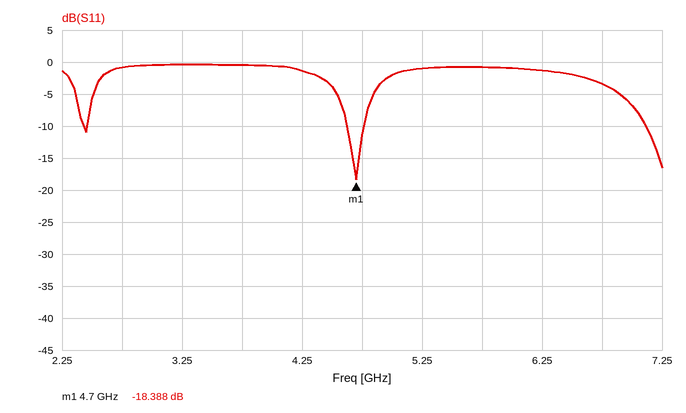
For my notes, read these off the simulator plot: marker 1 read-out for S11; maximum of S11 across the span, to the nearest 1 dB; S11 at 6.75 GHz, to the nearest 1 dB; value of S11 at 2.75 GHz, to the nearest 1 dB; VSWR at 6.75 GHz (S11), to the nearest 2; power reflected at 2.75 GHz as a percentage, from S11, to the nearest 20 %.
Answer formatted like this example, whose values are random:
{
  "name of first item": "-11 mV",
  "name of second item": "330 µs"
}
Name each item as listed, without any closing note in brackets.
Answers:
{
  "marker 1 read-out for S11": "-18.388 dB",
  "maximum of S11 across the span, to the nearest 1 dB": "0 dB",
  "S11 at 6.75 GHz, to the nearest 1 dB": "-3 dB",
  "value of S11 at 2.75 GHz, to the nearest 1 dB": "-1 dB",
  "VSWR at 6.75 GHz (S11), to the nearest 2": "6",
  "power reflected at 2.75 GHz as a percentage, from S11, to the nearest 20 %": "80 %"
}
